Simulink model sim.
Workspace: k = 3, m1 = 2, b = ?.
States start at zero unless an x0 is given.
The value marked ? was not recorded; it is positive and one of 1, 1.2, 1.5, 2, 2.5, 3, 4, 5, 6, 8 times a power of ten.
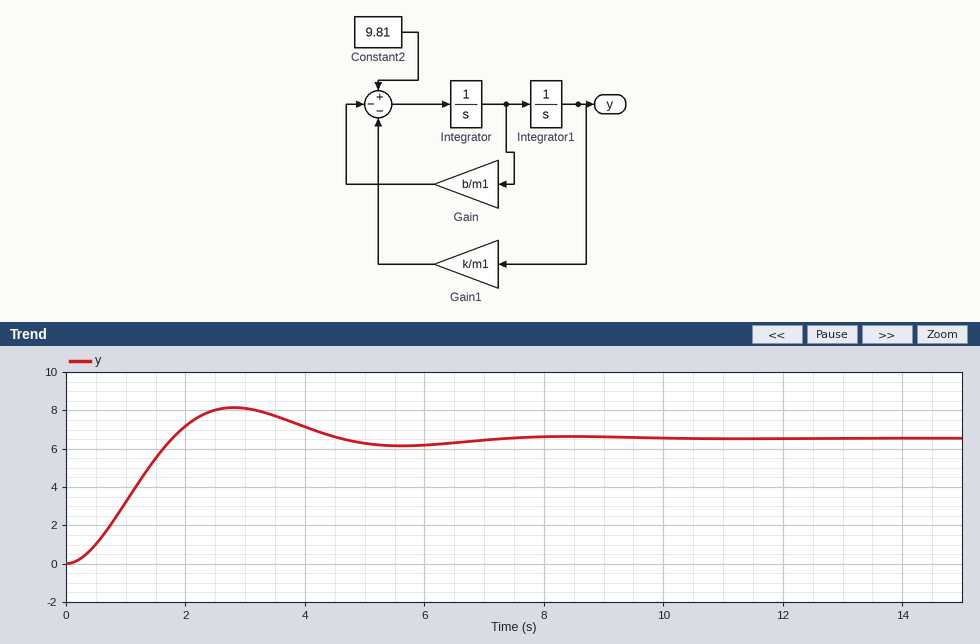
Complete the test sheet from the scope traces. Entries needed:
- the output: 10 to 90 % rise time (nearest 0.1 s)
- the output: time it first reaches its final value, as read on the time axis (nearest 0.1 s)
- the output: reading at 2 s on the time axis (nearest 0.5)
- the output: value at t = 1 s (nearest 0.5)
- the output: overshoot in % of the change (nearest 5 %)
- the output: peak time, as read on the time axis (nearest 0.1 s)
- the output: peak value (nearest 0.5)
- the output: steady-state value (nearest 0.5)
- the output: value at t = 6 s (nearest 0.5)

1.2 s
1.8 s
7.0
3.0
25 %
2.8 s
8.0
6.5
6.0
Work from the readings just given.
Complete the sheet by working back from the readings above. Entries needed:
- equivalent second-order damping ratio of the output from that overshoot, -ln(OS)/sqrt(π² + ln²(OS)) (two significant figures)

0.40
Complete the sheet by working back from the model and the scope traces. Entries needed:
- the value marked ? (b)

2
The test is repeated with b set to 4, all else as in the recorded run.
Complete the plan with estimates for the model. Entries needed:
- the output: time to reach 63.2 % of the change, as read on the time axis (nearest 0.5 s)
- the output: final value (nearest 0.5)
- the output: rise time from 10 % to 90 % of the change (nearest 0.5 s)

1.5 s
6.5
2.0 s
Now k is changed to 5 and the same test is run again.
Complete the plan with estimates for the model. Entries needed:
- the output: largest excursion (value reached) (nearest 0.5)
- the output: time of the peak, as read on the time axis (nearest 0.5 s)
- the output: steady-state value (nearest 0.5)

5.5
2.0 s
4.0
